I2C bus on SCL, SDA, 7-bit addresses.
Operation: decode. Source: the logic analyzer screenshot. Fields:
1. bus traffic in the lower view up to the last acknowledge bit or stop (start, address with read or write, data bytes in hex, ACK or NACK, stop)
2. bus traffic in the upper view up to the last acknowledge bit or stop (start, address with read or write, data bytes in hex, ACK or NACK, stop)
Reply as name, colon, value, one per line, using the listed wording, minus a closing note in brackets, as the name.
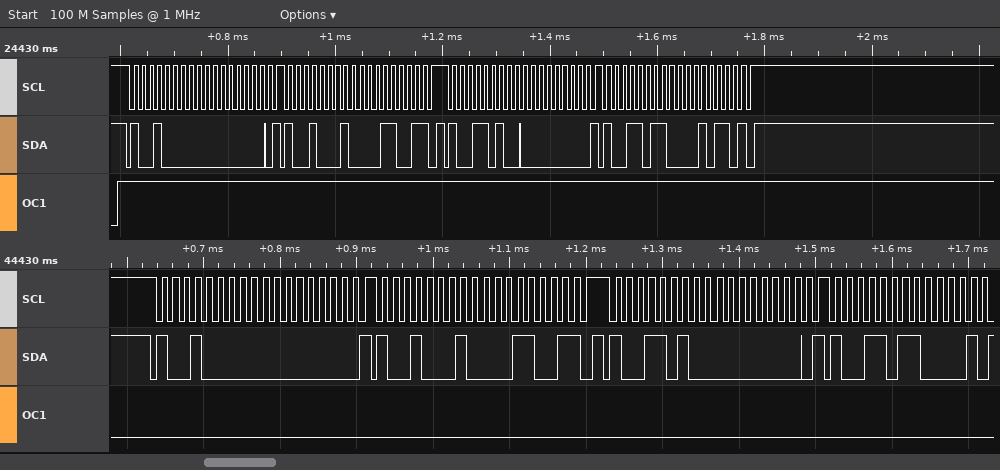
bus traffic in the lower view up to the last acknowledge bit or stop: start, address 48 write ACK, 00 ACK, repeated start, address 48 read ACK, 19 NACK, stop, start, address 4D write ACK, 00 ACK, repeated start, address 4D read ACK
bus traffic in the upper view up to the last acknowledge bit or stop: start, address 48 write ACK, 00 ACK, repeated start, address 48 read ACK, 19 NACK, stop, start, address 4D write ACK, 00 ACK, repeated start, address 4D read ACK, 16 NACK, stop
